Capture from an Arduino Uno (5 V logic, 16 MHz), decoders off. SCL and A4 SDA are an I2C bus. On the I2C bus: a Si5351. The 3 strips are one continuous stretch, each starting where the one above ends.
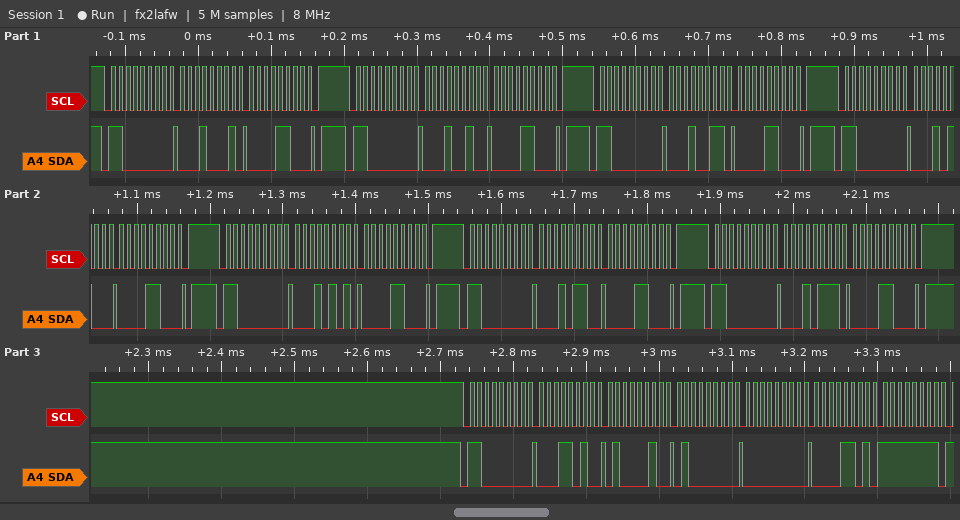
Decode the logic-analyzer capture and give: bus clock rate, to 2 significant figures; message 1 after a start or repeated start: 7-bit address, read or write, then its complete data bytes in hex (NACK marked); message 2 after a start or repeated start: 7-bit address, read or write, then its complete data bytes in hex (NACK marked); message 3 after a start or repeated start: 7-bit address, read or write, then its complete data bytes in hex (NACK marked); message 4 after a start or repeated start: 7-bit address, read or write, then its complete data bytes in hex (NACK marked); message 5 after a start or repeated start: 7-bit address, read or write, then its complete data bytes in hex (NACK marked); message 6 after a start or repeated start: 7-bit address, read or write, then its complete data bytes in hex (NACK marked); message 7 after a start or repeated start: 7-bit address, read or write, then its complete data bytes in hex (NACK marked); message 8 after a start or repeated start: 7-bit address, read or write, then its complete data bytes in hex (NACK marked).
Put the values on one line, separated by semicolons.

100 kHz; 0x60 write: 11 0C; 0x60 write: 12 0C; 0x60 write: 13 0C; 0x60 write: 14 0C; 0x60 write: 15 0C; 0x60 write: 16 0C; 0x60 write: 17 0C; 0x60 write: 1A 42 40 00 0D FF
